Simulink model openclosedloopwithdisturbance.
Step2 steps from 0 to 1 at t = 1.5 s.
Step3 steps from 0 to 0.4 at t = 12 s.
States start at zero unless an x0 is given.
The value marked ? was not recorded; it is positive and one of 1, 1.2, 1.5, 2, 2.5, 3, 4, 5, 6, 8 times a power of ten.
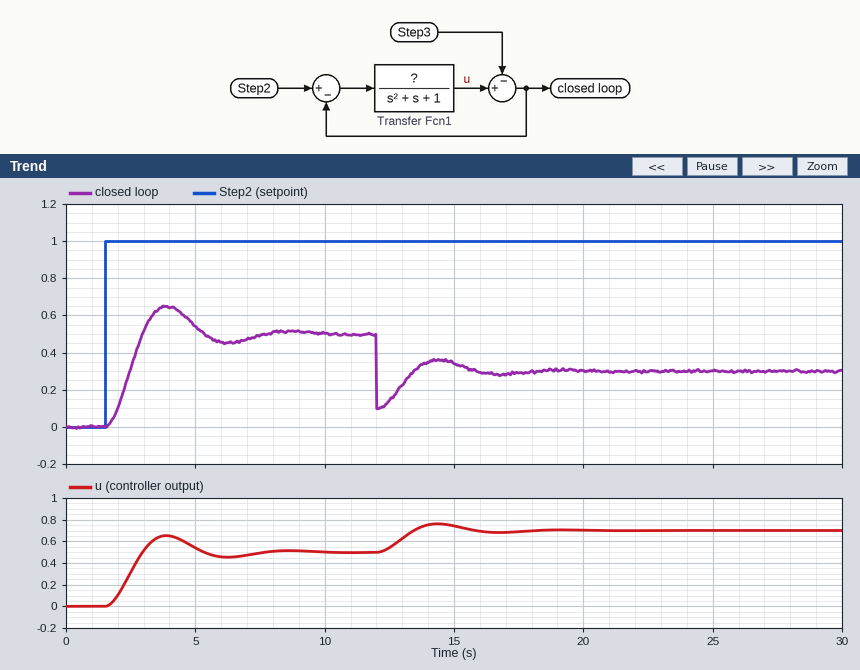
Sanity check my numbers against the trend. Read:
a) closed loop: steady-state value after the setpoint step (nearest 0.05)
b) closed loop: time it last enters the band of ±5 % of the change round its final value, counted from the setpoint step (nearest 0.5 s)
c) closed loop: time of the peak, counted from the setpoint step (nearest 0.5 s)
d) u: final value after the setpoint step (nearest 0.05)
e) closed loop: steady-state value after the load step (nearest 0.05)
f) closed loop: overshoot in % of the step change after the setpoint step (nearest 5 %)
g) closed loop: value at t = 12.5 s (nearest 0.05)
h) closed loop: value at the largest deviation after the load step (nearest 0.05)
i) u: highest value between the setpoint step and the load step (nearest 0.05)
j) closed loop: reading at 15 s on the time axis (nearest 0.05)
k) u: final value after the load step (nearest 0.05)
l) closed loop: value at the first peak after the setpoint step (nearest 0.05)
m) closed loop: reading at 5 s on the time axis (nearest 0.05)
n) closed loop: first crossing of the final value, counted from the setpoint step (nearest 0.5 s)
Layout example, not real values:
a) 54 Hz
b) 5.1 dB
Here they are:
a) 0.50
b) 5.5 s
c) 2.5 s
d) 0.50
e) 0.30
f) 30 %
g) 0.15
h) 0.10
i) 0.65
j) 0.35
k) 0.70
l) 0.65
m) 0.55
n) 1.5 s
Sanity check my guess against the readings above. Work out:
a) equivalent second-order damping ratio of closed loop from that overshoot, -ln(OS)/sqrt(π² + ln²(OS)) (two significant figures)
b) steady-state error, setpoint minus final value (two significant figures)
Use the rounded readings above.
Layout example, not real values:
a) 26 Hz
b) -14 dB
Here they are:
a) 0.36
b) 0.50
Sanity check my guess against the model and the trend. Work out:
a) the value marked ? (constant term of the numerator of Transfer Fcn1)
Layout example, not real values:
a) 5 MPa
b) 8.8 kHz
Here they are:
a) 1
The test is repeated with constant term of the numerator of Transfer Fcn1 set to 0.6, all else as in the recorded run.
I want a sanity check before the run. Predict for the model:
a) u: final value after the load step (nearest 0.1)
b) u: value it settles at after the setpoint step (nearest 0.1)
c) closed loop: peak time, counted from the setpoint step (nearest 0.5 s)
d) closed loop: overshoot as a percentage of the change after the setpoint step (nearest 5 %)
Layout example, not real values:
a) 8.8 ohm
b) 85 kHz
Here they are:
a) 0.5
b) 0.4
c) 2.5 s
d) 25 %
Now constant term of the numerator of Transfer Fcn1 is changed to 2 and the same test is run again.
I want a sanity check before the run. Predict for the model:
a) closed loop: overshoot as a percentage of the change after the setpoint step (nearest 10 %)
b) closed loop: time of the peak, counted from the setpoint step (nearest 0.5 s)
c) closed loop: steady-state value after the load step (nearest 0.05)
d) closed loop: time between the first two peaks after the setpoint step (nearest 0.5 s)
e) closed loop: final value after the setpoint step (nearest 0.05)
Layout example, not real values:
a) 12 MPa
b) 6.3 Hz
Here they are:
a) 40 %
b) 2.0 s
c) 0.55
d) 4.0 s
e) 0.65
